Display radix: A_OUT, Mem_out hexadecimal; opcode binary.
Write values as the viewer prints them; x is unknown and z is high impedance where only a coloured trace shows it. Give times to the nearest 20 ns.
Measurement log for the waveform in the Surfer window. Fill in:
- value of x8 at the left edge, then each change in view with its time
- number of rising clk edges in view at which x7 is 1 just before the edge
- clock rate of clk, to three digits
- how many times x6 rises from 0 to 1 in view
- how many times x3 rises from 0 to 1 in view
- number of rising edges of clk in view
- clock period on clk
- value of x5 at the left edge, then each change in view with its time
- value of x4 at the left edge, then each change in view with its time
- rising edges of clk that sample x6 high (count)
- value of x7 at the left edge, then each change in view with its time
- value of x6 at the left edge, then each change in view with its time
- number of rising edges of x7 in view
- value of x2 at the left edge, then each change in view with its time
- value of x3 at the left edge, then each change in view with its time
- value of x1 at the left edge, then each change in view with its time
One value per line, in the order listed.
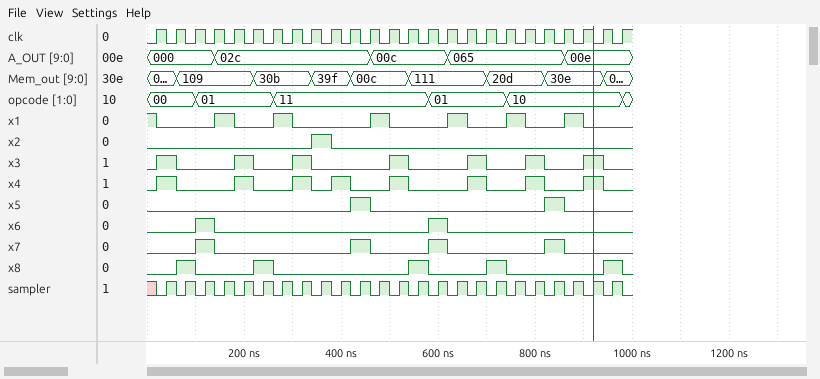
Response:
0, 1 at 60 ns, 0 at 100 ns, 1 at 220 ns, 0 at 260 ns, 1 at 540 ns, 0 at 580 ns, 1 at 700 ns, 0 at 740 ns, 1 at 940 ns, 0 at 980 ns
4
25.0 MHz
2
7
25
40 ns
0, 1 at 420 ns, 0 at 460 ns, 1 at 820 ns, 0 at 860 ns
0, 1 at 20 ns, 0 at 60 ns, 1 at 180 ns, 0 at 220 ns, 1 at 300 ns, 0 at 340 ns, 1 at 380 ns, 0 at 420 ns, 1 at 500 ns, 0 at 540 ns, 1 at 660 ns, 0 at 700 ns, 1 at 780 ns, 0 at 820 ns, 1 at 900 ns, 0 at 940 ns
2
0, 1 at 100 ns, 0 at 140 ns, 1 at 420 ns, 0 at 460 ns, 1 at 580 ns, 0 at 620 ns, 1 at 820 ns, 0 at 860 ns
0, 1 at 100 ns, 0 at 140 ns, 1 at 580 ns, 0 at 620 ns
4
0, 1 at 340 ns, 0 at 380 ns
0, 1 at 20 ns, 0 at 60 ns, 1 at 180 ns, 0 at 220 ns, 1 at 300 ns, 0 at 340 ns, 1 at 500 ns, 0 at 540 ns, 1 at 660 ns, 0 at 700 ns, 1 at 780 ns, 0 at 820 ns, 1 at 900 ns, 0 at 940 ns
1, 0 at 20 ns, 1 at 140 ns, 0 at 180 ns, 1 at 260 ns, 0 at 300 ns, 1 at 460 ns, 0 at 500 ns, 1 at 620 ns, 0 at 660 ns, 1 at 740 ns, 0 at 780 ns, 1 at 860 ns, 0 at 900 ns
